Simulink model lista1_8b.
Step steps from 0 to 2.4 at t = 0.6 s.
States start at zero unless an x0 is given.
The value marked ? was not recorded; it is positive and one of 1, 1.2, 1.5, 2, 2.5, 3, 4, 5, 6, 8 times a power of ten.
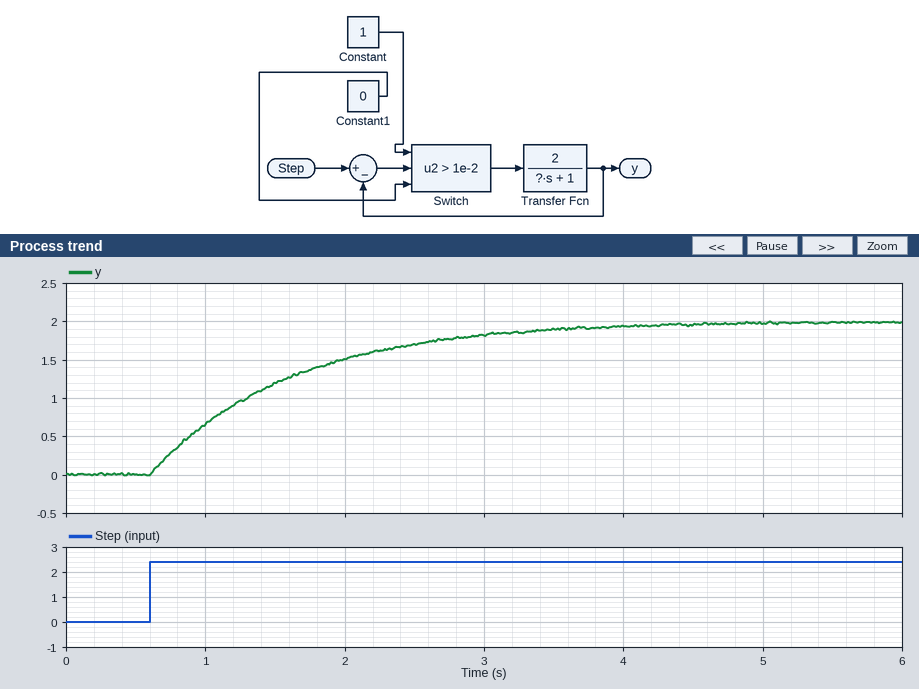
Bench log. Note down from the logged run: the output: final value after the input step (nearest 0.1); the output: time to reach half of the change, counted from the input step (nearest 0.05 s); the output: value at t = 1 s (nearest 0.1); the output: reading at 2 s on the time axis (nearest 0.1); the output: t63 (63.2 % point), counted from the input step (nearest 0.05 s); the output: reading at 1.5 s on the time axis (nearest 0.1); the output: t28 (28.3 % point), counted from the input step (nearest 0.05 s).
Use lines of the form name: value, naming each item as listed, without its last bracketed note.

the output: final value after the input step: 2.0
the output: time to reach half of the change, counted from the input step: 0.70 s
the output: value at t = 1 s: 0.7
the output: reading at 2 s on the time axis: 1.5
the output: t63 (63.2 % point), counted from the input step: 1.00 s
the output: reading at 1.5 s on the time axis: 1.2
the output: t28 (28.3 % point), counted from the input step: 0.35 s
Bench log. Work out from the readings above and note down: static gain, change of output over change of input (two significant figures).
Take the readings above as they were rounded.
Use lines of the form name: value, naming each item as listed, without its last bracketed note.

static gain, change of output over change of input: 0.83
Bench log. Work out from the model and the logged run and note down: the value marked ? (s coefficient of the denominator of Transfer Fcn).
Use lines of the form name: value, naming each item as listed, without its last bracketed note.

the value marked ?: 1
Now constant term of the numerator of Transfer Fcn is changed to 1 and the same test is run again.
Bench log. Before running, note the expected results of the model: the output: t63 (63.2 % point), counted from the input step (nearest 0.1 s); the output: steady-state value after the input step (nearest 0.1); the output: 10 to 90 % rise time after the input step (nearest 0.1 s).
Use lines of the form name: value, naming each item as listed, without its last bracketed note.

the output: t63 (63.2 % point), counted from the input step: 1.0 s
the output: steady-state value after the input step: 1.0
the output: 10 to 90 % rise time after the input step: 2.2 s
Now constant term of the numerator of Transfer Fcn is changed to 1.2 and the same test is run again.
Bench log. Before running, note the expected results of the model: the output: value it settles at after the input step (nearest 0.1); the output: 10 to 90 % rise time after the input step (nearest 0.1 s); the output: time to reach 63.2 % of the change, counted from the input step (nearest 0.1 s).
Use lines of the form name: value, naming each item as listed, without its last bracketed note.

the output: value it settles at after the input step: 1.2
the output: 10 to 90 % rise time after the input step: 2.2 s
the output: time to reach 63.2 % of the change, counted from the input step: 1.0 s
